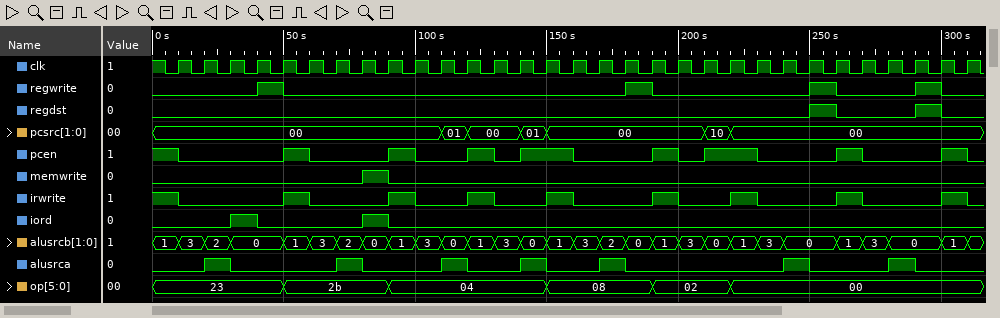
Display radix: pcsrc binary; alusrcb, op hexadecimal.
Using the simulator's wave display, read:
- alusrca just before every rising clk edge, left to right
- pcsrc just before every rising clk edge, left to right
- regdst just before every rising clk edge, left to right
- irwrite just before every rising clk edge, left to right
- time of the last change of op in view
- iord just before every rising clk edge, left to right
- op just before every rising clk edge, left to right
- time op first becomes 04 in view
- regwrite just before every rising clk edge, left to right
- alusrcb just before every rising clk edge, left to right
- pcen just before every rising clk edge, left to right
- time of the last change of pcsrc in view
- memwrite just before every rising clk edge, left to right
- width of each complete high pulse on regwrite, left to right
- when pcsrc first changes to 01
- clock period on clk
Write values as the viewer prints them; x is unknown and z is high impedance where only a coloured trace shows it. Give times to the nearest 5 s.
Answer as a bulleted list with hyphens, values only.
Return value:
- 0 0 1 0 0 0 0 1 0 0 0 1 0 0 1 0 0 1 0 0 0 0 0 0 1 0 0 0 1 0 0
- 00, 00, 00, 00, 00, 00, 00, 00, 00, 00, 00, 01, 00, 00, 01, 00, 00, 00, 00, 00, 00, 10, 00, 00, 00, 00, 00, 00, 00, 00, 00
- 0 0 0 0 0 0 0 0 0 0 0 0 0 0 0 0 0 0 0 0 0 0 0 0 0 1 0 0 0 1 0
- 1 0 0 0 0 1 0 0 0 1 0 0 1 0 0 1 0 0 0 1 0 0 1 0 0 0 1 0 0 0 1
- 220 s
- 0 0 0 1 0 0 0 0 1 0 0 0 0 0 0 0 0 0 0 0 0 0 0 0 0 0 0 0 0 0 0
- 23, 23, 23, 23, 23, 2b, 2b, 2b, 2b, 04, 04, 04, 04, 04, 04, 08, 08, 08, 08, 02, 02, 02, 00, 00, 00, 00, 00, 00, 00, 00, 00
- 90 s
- 0 0 0 0 1 0 0 0 0 0 0 0 0 0 0 0 0 0 1 0 0 0 0 0 0 1 0 0 0 1 0
- 1, 3, 2, 0, 0, 1, 3, 2, 0, 1, 3, 0, 1, 3, 0, 1, 3, 2, 0, 1, 3, 0, 1, 3, 0, 0, 1, 3, 0, 0, 1
- 1 0 0 0 0 1 0 0 0 1 0 0 1 0 1 1 0 0 0 1 0 1 1 0 0 0 1 0 0 0 1
- 220 s
- 0 0 0 0 0 0 0 0 1 0 0 0 0 0 0 0 0 0 0 0 0 0 0 0 0 0 0 0 0 0 0
- 10 s, 10 s, 10 s, 10 s
- 110 s
- 10 s
